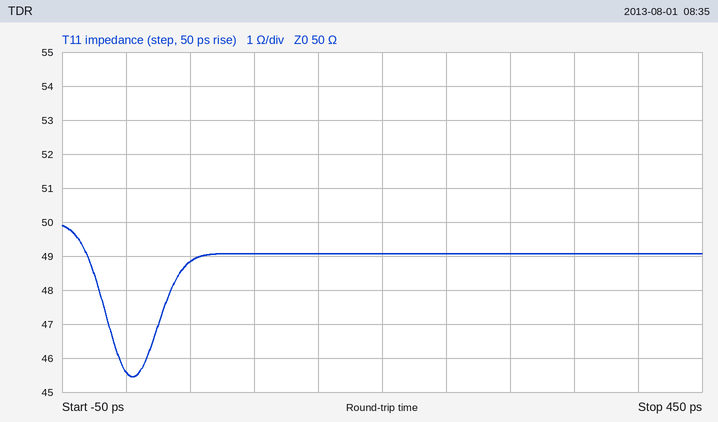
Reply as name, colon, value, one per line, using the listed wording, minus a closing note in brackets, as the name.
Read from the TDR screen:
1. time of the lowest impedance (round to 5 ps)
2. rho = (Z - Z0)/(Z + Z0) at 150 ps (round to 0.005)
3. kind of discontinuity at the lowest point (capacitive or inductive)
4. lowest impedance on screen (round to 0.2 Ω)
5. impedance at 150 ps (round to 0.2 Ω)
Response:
time of the lowest impedance: 5 ps
rho = (Z - Z0)/(Z + Z0) at 150 ps: -0.010
kind of discontinuity at the lowest point: capacitive
lowest impedance on screen: 45.4 Ω
impedance at 150 ps: 49.0 Ω
